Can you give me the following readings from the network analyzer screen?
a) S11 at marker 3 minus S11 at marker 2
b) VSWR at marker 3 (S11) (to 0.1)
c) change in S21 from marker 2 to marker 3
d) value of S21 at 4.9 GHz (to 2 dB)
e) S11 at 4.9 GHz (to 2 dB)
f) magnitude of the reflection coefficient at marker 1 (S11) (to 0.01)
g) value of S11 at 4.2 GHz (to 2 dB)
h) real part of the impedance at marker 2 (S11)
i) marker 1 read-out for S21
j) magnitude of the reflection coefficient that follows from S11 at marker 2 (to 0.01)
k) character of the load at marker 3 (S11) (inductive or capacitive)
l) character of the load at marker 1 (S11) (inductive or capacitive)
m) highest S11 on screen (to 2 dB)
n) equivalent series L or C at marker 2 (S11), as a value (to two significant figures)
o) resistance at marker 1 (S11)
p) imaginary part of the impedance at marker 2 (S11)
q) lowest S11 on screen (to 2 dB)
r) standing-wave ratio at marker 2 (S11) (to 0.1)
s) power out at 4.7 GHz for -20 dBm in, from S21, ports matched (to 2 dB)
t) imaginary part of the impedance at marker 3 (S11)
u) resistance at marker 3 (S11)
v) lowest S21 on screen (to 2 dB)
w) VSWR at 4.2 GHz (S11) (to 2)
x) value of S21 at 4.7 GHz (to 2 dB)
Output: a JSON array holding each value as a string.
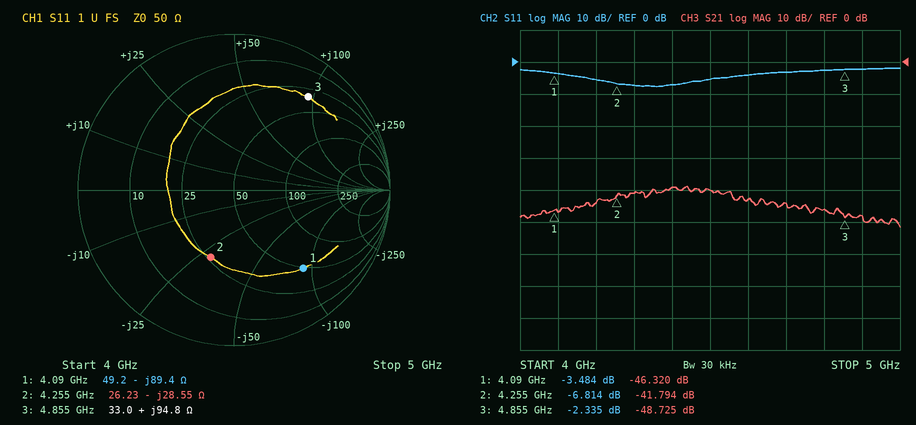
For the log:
["4.479 dB", "7.5", "-6.931 dB", "-48 dB", "-2 dB", "0.67", "-6 dB", "26.23 Ω", "-46.320 dB", "0.46", "inductive", "capacitive", "-2 dB", "1.3 pF", "49.2 Ω", "-28.55 Ω", "-8 dB", "2.7", "-64 dBm", "+94.8 Ω", "33.0 Ω", "-52 dB", "4", "-44 dB"]
